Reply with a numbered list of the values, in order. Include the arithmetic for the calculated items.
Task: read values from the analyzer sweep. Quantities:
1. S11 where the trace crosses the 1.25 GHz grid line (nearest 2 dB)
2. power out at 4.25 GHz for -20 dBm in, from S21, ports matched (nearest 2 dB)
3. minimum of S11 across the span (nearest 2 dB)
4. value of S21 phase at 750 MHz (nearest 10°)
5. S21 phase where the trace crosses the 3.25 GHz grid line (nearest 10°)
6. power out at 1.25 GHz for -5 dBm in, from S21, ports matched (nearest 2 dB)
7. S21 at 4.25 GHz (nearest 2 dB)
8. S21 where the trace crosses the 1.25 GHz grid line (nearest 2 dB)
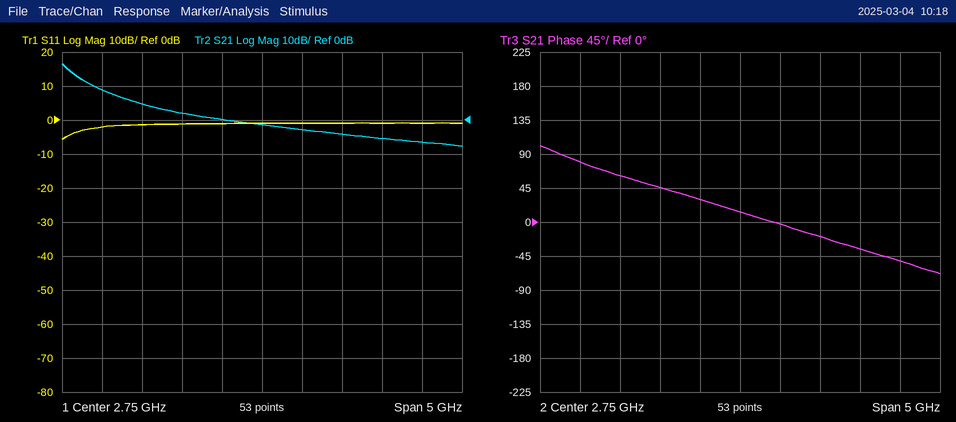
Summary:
1. -2 dB
2. -20 dBm + (-6 dB) = -26 dBm
3. -6 dB
4. 80°
5. 0°
6. -5 dBm + (4 dB) = 0 dBm
7. -6 dB
8. 4 dB
